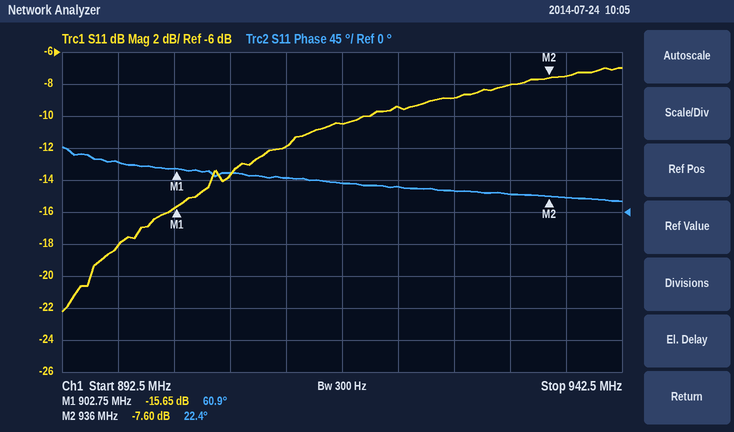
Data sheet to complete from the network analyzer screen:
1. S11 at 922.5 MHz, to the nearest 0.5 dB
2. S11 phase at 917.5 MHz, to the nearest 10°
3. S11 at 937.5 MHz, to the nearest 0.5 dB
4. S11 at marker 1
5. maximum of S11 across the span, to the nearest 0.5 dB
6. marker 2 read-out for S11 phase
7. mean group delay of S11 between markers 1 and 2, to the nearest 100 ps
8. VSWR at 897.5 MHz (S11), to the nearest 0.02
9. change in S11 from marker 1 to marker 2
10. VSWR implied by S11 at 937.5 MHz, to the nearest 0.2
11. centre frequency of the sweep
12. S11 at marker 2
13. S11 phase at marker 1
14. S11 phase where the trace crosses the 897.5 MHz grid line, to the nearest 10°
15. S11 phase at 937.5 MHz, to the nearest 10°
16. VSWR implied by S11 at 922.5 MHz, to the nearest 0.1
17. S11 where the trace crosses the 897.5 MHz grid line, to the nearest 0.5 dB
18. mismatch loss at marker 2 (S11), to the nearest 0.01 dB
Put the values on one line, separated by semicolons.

-9.5 dB; 40°; -7.5 dB; -15.65 dB; -7.0 dB; 22.4°; 3.2 ns; 1.28; 8.05 dB; 2.4; 917.5 MHz; -7.60 dB; 60.9°; 70°; 20°; 2.0; -18.0 dB; 0.83 dB
